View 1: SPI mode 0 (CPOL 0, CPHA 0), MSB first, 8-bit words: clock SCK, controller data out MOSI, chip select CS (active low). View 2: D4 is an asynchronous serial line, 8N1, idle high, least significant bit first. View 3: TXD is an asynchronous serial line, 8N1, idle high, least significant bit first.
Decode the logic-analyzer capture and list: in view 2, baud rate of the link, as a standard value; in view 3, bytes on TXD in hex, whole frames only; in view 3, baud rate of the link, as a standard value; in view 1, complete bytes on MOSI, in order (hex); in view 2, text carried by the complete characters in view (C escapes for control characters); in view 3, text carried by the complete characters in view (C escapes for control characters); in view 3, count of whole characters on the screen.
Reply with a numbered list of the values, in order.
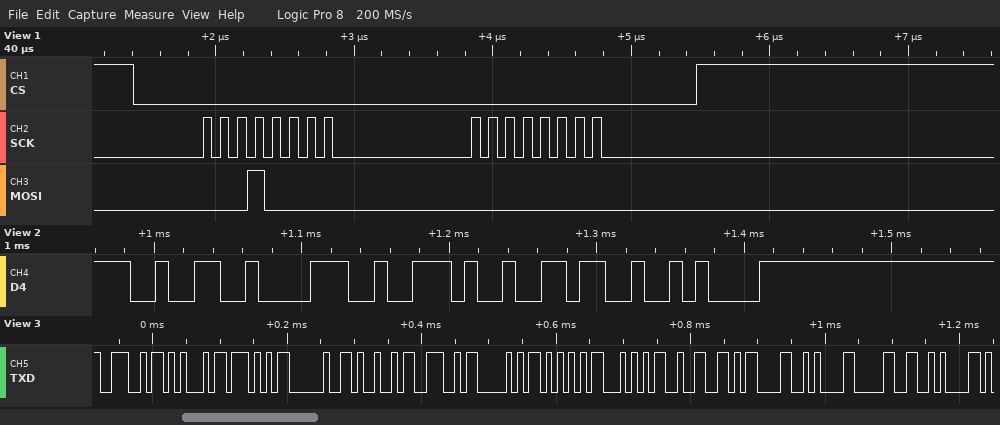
1. 115200 baud
2. 4E 45 57 20 49 4E 50 55 54 32 0D 0A 30 0A
3. 115200 baud
4. 10 00
5. "28.6\n"
6. "NEW INPUT2\r\n0\n"
7. 14
